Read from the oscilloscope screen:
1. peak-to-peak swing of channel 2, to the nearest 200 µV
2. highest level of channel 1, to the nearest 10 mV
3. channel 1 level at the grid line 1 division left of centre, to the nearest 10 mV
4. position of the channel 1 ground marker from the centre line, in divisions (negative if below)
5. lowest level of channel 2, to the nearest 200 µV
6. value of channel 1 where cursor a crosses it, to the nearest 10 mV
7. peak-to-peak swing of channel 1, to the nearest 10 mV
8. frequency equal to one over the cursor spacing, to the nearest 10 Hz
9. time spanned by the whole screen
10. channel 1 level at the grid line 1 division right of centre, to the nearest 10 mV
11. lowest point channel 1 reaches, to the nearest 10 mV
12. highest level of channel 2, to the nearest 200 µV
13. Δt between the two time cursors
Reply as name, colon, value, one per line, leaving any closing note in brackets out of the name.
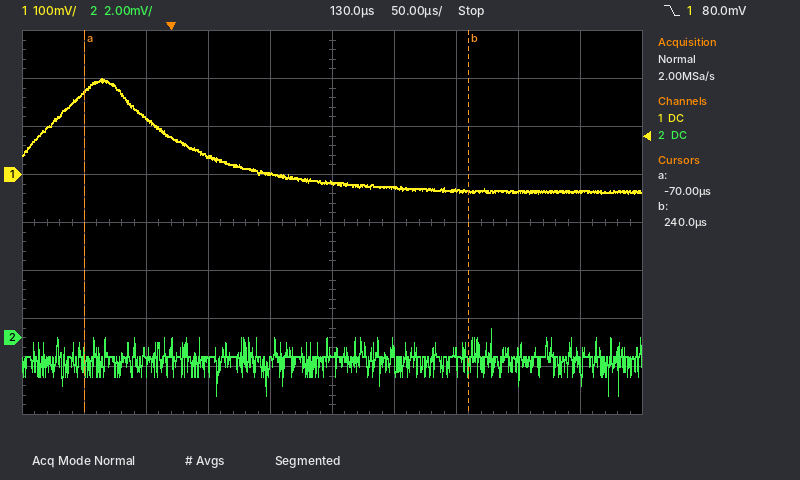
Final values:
peak-to-peak swing of channel 2, to the nearest 200 µV: 2.8 mV
highest level of channel 1, to the nearest 10 mV: 200 mV
channel 1 level at the grid line 1 division left of centre, to the nearest 10 mV: 0 mV
position of the channel 1 ground marker from the centre line, in divisions: +1.0 div
lowest level of channel 2, to the nearest 200 µV: -2.4 mV
value of channel 1 where cursor a crosses it, to the nearest 10 mV: 170 mV
peak-to-peak swing of channel 1, to the nearest 10 mV: 240 mV
frequency equal to one over the cursor spacing, to the nearest 10 Hz: 3.23 kHz
time spanned by the whole screen: 500 µs
channel 1 level at the grid line 1 division right of centre, to the nearest 10 mV: -30 mV
lowest point channel 1 reaches, to the nearest 10 mV: -40 mV
highest level of channel 2, to the nearest 200 µV: 400 µV
Δt between the two time cursors: 310 µs
